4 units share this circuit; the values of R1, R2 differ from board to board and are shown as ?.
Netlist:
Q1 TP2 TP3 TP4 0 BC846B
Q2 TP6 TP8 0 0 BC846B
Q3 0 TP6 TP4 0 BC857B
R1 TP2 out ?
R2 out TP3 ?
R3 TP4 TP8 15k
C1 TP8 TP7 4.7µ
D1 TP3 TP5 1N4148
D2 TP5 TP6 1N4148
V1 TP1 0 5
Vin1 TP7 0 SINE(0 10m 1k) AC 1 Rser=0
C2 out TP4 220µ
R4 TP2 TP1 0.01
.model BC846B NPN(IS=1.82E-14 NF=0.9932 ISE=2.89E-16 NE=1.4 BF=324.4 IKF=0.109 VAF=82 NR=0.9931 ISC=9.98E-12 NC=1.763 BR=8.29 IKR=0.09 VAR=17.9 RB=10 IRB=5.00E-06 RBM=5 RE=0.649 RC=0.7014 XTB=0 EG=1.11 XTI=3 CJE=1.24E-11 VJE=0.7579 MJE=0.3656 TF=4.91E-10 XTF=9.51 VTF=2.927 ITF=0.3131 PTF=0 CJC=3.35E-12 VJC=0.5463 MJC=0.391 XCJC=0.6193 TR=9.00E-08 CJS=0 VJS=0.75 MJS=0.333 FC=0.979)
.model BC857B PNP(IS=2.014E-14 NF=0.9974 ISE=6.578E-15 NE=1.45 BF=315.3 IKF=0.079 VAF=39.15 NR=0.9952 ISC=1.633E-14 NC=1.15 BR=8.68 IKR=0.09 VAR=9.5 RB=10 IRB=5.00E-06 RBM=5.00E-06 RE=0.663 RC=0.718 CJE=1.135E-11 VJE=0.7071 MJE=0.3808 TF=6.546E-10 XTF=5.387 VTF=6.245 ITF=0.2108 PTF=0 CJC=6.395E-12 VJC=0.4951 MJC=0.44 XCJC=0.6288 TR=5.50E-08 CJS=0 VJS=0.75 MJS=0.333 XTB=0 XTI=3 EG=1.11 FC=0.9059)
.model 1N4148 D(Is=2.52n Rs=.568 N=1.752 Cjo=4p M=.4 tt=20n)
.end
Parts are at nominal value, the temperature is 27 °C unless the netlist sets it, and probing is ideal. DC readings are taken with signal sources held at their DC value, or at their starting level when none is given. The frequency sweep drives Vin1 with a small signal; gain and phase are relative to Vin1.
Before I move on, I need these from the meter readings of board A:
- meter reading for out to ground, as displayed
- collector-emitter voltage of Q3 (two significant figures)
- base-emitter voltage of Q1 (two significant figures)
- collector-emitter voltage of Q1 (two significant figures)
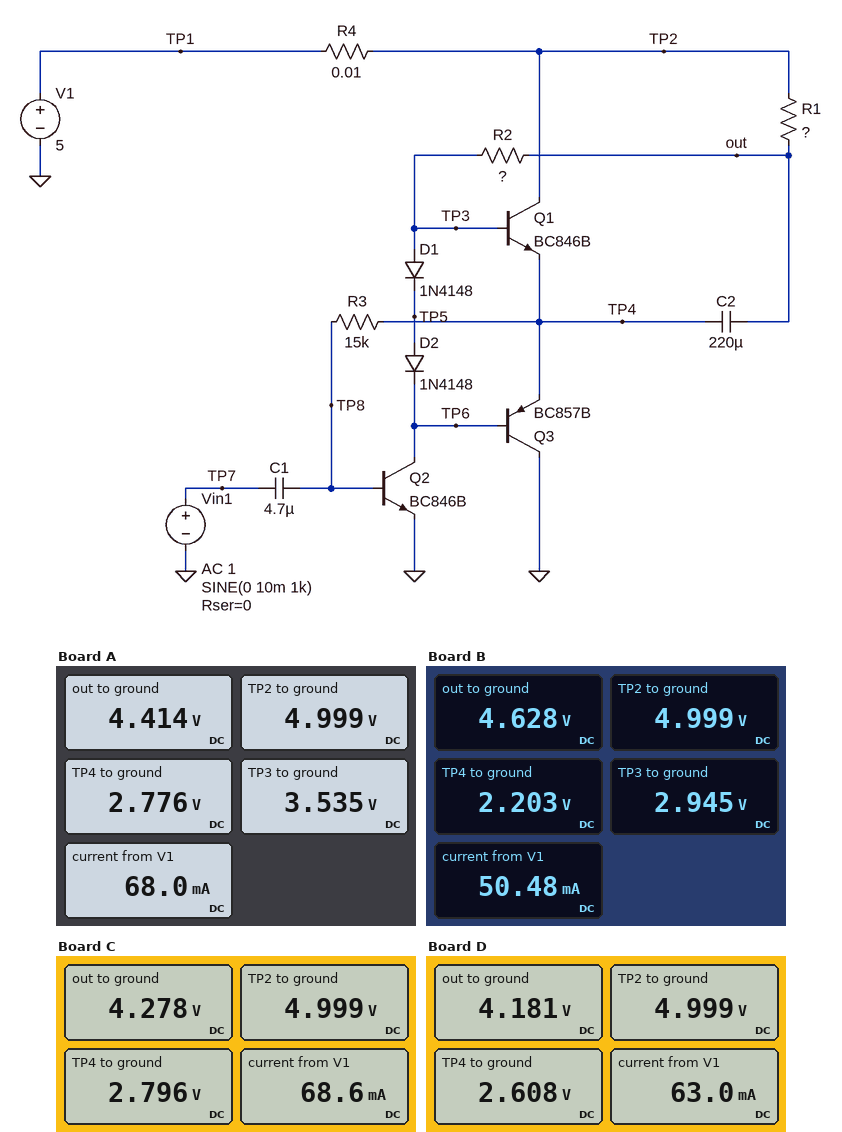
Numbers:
4.414 V
-2.8 V
760 mV
2.2 V
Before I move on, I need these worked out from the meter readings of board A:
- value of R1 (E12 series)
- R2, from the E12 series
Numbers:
18 Ω
27 Ω
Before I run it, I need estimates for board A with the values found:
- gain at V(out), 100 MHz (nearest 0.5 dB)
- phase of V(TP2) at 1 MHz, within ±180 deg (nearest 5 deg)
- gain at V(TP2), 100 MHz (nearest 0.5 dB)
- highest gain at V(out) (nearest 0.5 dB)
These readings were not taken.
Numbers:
18.5 dB
170 deg
-47.5 dB
49.0 dB
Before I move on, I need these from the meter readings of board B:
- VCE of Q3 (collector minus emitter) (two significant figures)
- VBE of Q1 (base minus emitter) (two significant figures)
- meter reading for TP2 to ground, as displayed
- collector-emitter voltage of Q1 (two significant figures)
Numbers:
-2.2 V
740 mV
4.999 V
2.8 V
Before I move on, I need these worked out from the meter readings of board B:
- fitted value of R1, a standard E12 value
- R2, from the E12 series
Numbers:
15 Ω
68 Ω
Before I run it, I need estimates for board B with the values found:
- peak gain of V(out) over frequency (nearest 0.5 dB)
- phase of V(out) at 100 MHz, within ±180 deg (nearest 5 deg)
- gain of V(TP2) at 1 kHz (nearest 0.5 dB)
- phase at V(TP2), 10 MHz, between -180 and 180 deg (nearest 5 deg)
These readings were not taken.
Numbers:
51.0 dB
60 deg
-22.5 dB
110 deg
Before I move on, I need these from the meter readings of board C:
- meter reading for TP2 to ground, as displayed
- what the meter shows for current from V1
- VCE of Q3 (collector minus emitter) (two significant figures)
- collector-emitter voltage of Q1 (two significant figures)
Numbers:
4.999 V
68.6 mA
-2.8 V
2.2 V
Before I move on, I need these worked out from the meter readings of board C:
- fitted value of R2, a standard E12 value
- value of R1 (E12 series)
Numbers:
22 Ω
22 Ω
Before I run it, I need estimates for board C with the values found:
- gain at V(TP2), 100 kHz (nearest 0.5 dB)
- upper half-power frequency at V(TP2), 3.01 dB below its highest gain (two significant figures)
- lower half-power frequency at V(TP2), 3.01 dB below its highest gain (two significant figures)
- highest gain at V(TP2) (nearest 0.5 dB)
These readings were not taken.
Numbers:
-22.5 dB
5.5 MHz
1.4 kHz
-22.5 dB
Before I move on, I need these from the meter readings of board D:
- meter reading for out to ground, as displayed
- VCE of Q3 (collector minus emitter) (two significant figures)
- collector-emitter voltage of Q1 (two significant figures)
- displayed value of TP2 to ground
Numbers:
4.181 V
-2.6 V
2.4 V
4.999 V
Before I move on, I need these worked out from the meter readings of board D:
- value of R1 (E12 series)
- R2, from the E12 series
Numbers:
27 Ω
27 Ω
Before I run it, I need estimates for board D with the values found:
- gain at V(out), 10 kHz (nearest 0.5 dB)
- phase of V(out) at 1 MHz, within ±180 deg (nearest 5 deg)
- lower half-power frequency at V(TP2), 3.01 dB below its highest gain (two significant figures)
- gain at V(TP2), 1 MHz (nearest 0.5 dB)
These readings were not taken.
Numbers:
51.5 dB
170 deg
1.5 kHz
-22.5 dB
